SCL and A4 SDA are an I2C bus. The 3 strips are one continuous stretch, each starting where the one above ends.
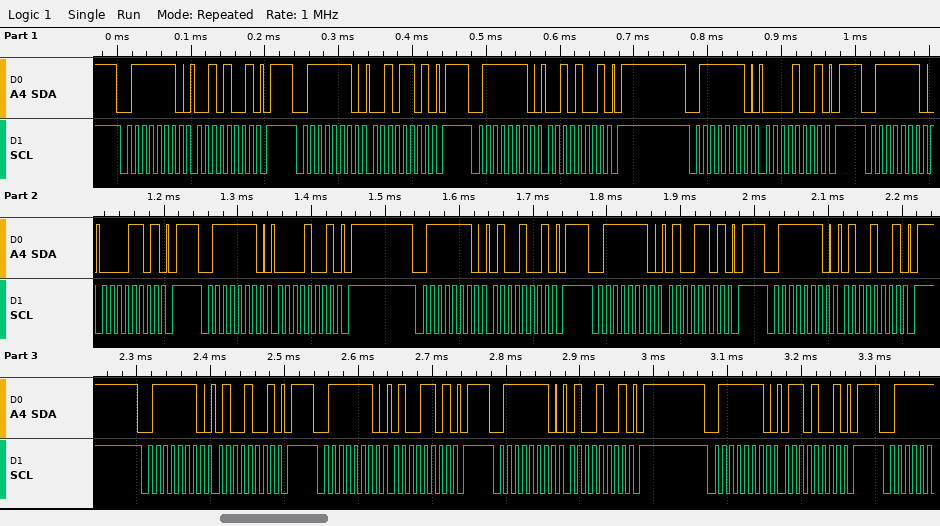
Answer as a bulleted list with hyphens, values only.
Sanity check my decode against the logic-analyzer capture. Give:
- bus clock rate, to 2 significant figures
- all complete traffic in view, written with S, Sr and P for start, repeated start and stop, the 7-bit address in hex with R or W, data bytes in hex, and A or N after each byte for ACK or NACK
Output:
- 100 kHz
- S 3FW A 29 A P S 3FW A 2D A P S 3FW A 29 A P S 3FW A 09 A P S 3FW A 0D A P S 3FW A 09 A P S 3FW A 49 A P S 3FW A 4D A P S 3FW A 49 A P S 3FW A 49 A P S 3FW A 4D A P S 3FW A 49 A P S 3FW A 69 A P
